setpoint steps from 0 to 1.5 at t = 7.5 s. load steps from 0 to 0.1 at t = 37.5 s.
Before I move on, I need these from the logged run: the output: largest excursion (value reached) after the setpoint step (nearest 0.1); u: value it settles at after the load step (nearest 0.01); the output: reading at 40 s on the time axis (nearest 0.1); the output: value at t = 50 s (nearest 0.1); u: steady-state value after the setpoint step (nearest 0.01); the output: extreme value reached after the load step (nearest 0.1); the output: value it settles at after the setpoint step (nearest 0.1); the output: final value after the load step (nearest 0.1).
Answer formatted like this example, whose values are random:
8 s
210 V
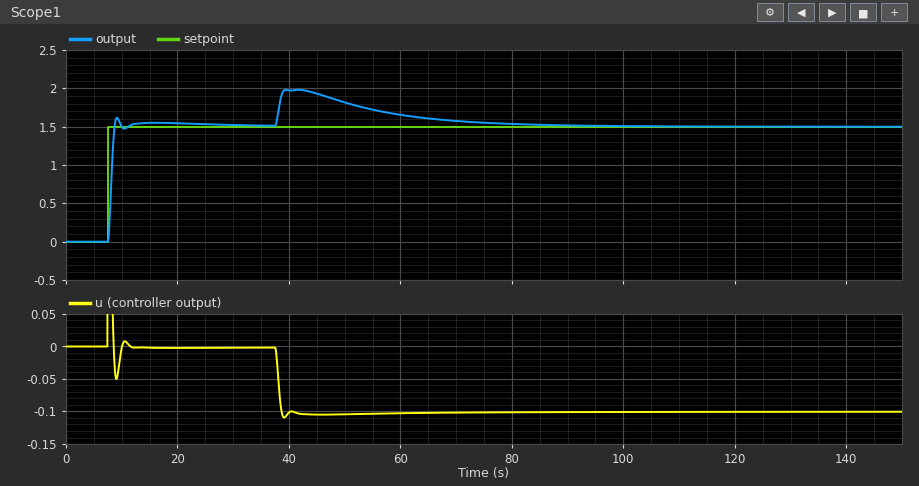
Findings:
1.6
-0.10
2.0
1.8
0.00
2.0
1.5
1.5
